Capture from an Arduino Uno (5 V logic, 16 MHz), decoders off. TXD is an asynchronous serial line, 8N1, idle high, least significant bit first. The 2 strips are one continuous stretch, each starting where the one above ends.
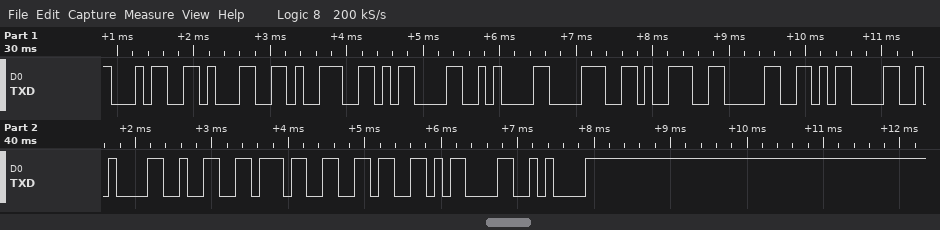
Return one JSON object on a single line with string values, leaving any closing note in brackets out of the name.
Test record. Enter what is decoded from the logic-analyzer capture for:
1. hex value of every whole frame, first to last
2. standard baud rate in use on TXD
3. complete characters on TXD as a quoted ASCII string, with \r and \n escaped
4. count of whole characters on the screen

{"hex value of every whole frame, first to last": "0x34 0x31 0x39 0x0D 0x0A 0x38 0x39 0x30 0x0D 0x0A 0x32 0x37 0x36 0x0D 0x0A", "standard baud rate in use on TXD": "9600 baud", "complete characters on TXD as a quoted ASCII string, with \\r and \\n escaped": "\"419\\r\\n890\\r\\n276\\r\\n\"", "count of whole characters on the screen": "15"}
